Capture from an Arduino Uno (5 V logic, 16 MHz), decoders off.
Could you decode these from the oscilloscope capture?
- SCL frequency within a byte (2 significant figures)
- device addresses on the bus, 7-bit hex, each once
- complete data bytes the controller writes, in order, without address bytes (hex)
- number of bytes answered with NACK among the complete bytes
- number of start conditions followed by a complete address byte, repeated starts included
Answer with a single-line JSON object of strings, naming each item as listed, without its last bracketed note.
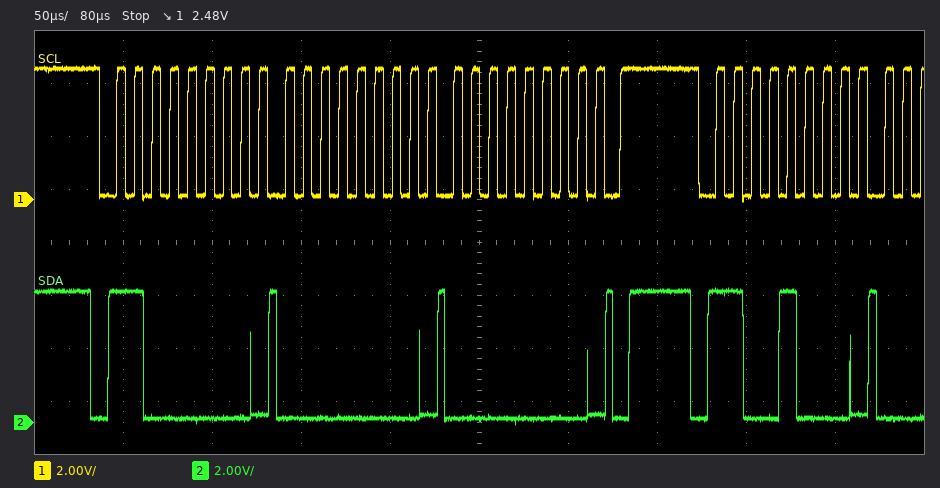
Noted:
{"SCL frequency within a byte": "100 kHz", "device addresses on the bus, 7-bit hex, each once": "0x60 0x64", "complete data bytes the controller writes, in order, without address bytes": "00 00", "number of bytes answered with NACK among the complete bytes": "0", "number of start conditions followed by a complete address byte, repeated starts included": "2"}
